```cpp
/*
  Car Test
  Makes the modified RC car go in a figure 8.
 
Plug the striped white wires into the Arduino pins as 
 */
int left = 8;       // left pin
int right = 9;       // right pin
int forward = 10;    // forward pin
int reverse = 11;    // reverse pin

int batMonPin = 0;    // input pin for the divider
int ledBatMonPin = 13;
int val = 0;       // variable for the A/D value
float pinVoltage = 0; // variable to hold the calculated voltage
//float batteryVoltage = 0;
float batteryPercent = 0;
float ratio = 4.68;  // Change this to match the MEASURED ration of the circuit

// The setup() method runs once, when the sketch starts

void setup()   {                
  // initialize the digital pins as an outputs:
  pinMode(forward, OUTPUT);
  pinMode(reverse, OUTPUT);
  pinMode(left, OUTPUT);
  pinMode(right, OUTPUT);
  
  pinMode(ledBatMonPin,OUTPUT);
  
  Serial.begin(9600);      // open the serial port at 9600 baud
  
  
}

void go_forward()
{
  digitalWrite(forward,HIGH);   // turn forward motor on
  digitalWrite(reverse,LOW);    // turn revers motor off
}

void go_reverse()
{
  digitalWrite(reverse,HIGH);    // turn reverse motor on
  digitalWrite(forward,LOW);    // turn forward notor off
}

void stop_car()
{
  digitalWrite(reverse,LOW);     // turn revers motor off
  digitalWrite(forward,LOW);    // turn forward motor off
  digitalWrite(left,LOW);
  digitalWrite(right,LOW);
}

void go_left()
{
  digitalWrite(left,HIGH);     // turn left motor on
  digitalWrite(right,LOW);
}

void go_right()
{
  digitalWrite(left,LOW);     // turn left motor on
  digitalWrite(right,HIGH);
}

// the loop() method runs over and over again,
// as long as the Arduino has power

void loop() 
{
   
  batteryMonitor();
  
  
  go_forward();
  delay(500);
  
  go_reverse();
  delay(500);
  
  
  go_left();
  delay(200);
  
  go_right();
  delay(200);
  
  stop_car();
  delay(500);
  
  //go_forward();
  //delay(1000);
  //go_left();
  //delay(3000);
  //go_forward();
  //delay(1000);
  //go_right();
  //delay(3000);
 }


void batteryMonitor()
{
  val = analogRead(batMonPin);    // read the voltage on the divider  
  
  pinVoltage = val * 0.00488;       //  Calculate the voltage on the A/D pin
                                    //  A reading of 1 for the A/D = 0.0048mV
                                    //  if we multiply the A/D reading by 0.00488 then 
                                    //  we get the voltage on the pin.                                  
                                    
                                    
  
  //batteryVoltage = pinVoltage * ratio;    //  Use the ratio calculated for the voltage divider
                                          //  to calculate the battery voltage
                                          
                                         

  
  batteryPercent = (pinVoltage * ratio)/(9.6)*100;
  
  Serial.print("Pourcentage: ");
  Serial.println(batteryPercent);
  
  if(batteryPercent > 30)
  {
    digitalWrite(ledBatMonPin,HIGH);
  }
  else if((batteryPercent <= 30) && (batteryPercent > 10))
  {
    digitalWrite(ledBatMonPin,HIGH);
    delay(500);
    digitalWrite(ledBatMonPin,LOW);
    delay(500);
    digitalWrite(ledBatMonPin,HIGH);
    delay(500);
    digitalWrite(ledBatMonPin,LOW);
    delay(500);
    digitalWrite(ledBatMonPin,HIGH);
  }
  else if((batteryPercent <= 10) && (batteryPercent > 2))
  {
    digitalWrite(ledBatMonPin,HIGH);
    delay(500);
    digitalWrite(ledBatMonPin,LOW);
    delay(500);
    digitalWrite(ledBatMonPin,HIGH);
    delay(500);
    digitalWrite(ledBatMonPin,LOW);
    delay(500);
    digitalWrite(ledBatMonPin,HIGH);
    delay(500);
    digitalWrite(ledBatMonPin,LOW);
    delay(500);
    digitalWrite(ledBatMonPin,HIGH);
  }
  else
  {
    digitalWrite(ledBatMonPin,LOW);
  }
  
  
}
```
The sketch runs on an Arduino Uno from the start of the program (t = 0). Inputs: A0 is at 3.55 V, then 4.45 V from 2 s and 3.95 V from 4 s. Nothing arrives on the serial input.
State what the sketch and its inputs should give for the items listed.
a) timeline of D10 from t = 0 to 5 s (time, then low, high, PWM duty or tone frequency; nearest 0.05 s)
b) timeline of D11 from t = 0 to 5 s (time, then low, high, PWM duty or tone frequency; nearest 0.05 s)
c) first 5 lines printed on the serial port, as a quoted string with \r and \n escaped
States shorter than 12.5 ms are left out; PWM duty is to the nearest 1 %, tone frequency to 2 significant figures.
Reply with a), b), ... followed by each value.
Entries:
a) 0 s high; 0.5 s low; 1.9 s high; 2.4 s low; 3.8 s high; 4.3 s low
b) 0 s low; 0.5 s high; 1.4 s low; 2.4 s high; 3.3 s low; 4.3 s high
c) "Pourcentage: 172.95\r\nPourcentage: 172.95\r\nPourcentage: 216.73\r\nPourcentage: 192.22\r\nPourcentage: 192.22\r\n"
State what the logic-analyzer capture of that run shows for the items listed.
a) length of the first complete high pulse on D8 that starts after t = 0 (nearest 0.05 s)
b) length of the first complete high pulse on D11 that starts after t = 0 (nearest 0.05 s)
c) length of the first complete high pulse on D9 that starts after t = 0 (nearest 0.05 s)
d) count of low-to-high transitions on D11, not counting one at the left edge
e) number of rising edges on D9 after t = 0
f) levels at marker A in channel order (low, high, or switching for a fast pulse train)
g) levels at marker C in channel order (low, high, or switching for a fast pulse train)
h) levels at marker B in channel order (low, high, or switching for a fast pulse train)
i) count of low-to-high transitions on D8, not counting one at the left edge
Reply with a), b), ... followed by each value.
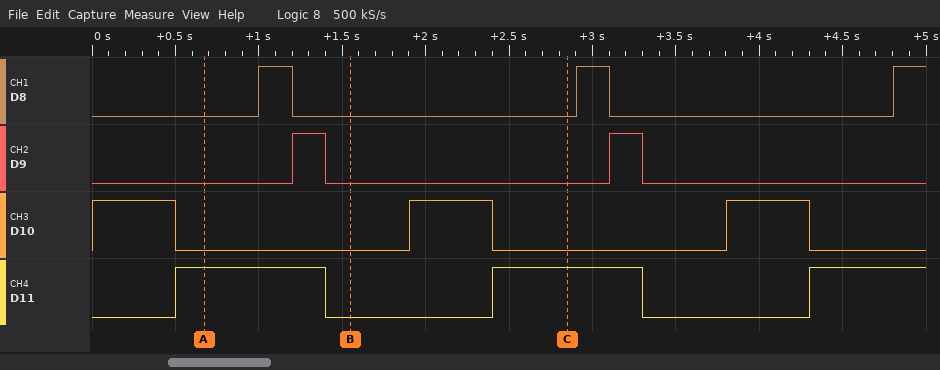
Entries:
a) 0.20 s
b) 0.90 s
c) 0.20 s
d) 3
e) 2
f) D8 low, D9 low, D10 low, D11 high
g) D8 low, D9 low, D10 low, D11 high
h) D8 low, D9 low, D10 low, D11 low
i) 3
